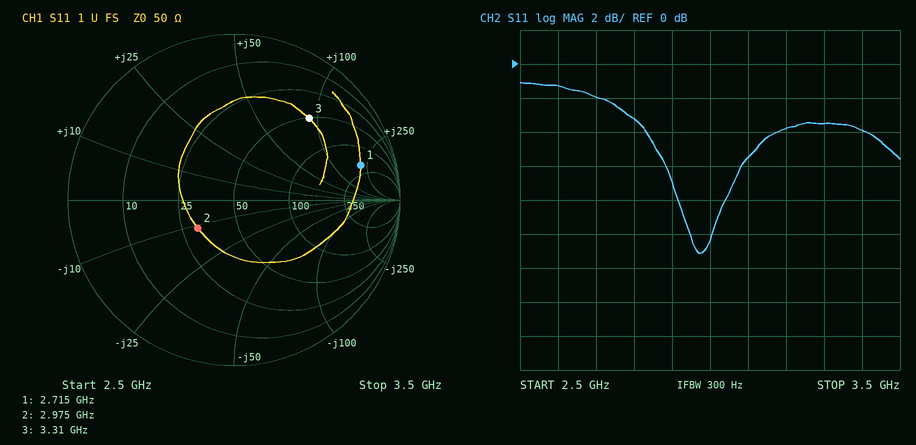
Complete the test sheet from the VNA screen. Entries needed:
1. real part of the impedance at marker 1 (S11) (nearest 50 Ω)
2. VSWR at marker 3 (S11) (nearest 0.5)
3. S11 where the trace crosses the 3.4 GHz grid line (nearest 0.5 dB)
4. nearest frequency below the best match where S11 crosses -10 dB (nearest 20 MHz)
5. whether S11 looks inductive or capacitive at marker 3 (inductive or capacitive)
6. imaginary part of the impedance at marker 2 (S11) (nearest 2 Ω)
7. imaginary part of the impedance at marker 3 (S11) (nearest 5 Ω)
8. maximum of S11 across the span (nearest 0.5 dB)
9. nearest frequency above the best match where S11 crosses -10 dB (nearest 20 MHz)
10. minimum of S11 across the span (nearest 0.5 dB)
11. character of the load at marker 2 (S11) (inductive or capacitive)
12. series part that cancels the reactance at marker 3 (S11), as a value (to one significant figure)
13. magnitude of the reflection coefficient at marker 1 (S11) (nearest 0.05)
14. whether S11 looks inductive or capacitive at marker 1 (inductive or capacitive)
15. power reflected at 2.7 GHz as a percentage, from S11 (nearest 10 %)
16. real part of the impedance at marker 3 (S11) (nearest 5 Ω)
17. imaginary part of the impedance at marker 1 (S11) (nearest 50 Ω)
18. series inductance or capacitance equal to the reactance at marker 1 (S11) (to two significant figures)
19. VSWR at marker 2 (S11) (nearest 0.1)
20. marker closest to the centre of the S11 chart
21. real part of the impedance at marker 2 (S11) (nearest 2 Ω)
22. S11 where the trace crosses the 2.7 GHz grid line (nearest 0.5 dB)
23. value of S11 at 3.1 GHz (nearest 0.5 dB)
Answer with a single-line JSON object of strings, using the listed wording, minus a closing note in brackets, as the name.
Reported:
{"real part of the impedance at marker 1 (S11)": "200 Ω", "VSWR at marker 3 (S11)": "5.0", "S11 where the trace crosses the 3.4 GHz grid line": "-4.0 dB", "nearest frequency below the best match where S11 crosses -10 dB": "2.94 GHz", "whether S11 looks inductive or capacitive at marker 3": "inductive", "imaginary part of the impedance at marker 2 (S11)": "-12 Ω", "imaginary part of the impedance at marker 3 (S11)": "+90 Ω", "maximum of S11 across the span": "-1.0 dB", "nearest frequency above the best match where S11 crosses -10 dB": "3.00 GHz", "minimum of S11 across the span": "-11.0 dB", "character of the load at marker 2 (S11)": "capacitive", "series part that cancels the reactance at marker 3 (S11), as a value": "500 fF", "magnitude of the reflection coefficient at marker 1 (S11)": "0.80", "whether S11 looks inductive or capacitive at marker 1": "inductive", "power reflected at 2.7 GHz as a percentage, from S11": "60 %", "real part of the impedance at marker 3 (S11)": "50 Ω", "imaginary part of the impedance at marker 1 (S11)": "+200 Ω", "series inductance or capacitance equal to the reactance at marker 1 (S11)": "12 nH", "VSWR at marker 2 (S11)": "1.8", "marker closest to the centre of the S11 chart": "marker 2", "real part of the impedance at marker 2 (S11)": "30 Ω", "S11 where the trace crosses the 2.7 GHz grid line": "-2.0 dB", "value of S11 at 3.1 GHz": "-5.5 dB"}
